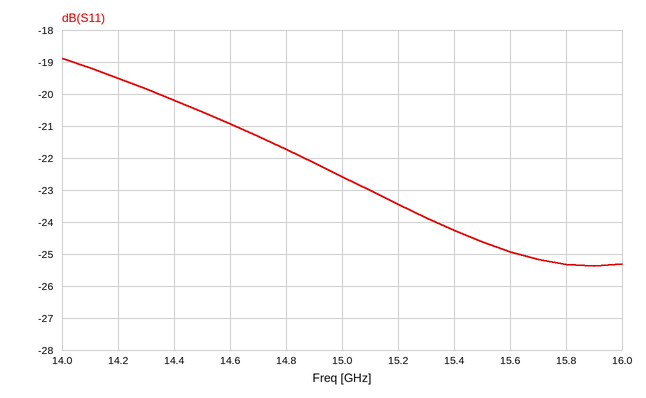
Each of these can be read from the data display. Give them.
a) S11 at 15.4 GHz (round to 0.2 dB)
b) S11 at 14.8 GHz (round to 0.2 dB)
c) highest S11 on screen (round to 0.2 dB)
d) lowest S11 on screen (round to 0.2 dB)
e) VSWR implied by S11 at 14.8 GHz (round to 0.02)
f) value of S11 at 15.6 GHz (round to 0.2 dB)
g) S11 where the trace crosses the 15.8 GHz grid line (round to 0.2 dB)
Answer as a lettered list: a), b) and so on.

a) -24.2 dB
b) -21.8 dB
c) -18.8 dB
d) -25.4 dB
e) 1.18
f) -25.0 dB
g) -25.4 dB
